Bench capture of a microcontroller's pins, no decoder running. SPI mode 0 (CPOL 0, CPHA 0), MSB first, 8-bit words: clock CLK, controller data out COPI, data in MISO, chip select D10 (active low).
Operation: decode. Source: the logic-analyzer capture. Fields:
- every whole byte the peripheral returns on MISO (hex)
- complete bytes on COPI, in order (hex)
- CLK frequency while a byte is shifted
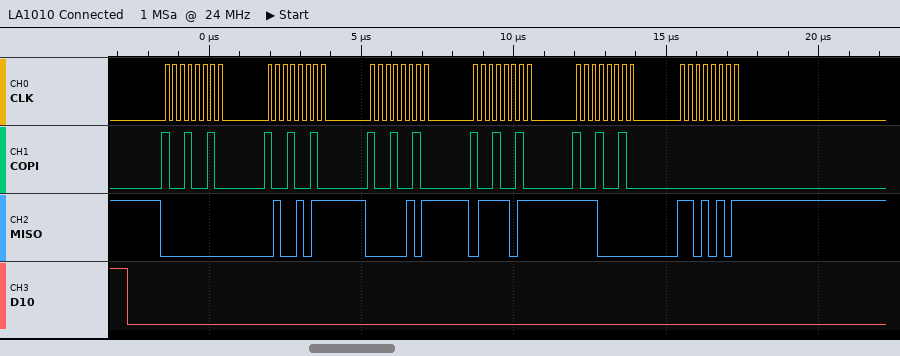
00 4B 05 7B E0 D5
92 92 92 92 92 00
4 MHz
